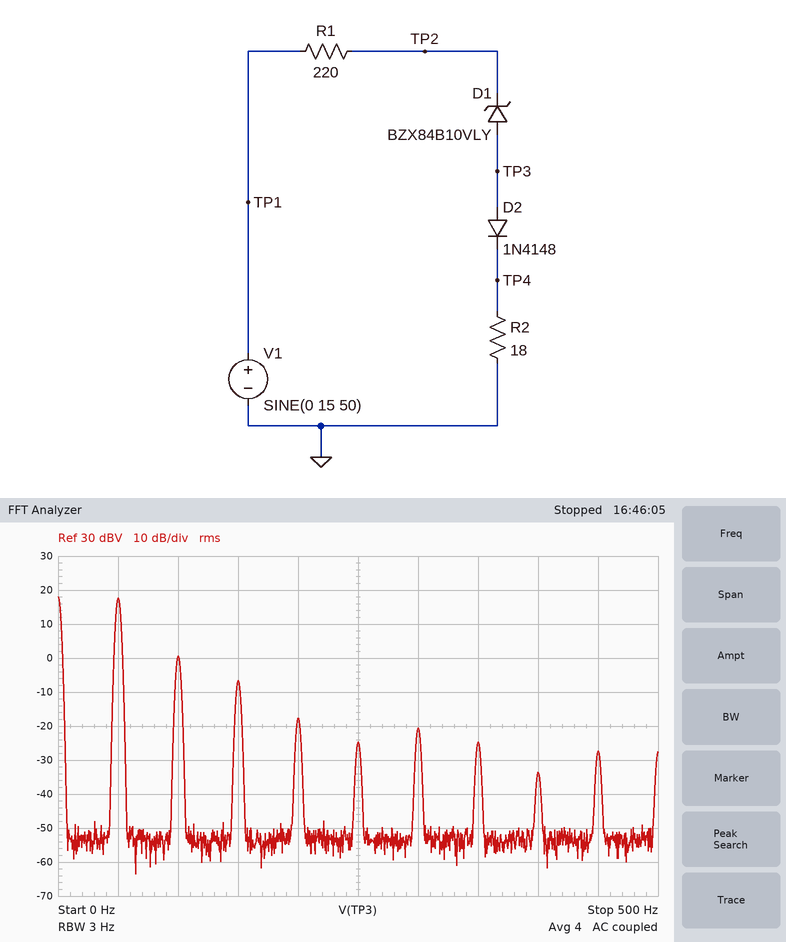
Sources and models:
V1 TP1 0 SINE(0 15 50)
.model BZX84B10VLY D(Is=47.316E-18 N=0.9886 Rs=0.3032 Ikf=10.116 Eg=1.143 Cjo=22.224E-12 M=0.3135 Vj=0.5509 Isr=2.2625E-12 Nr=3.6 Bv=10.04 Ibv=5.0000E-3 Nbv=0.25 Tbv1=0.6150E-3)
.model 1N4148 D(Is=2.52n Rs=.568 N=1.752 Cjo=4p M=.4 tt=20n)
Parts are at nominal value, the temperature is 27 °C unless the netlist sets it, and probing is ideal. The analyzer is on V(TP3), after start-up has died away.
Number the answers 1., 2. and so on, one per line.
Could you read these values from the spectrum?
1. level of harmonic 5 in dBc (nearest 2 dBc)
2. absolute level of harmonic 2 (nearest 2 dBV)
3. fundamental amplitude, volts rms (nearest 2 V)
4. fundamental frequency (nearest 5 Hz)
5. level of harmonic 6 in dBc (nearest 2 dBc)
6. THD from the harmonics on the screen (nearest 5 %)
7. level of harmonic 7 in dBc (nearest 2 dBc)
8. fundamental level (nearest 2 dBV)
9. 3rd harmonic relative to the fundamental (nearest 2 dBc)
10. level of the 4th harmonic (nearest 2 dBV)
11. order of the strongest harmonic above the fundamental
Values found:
1. -42 dBc
2. 0 dBV
3. 8 V
4. 50 Hz
5. -38 dBc
6. 15 %
7. -42 dBc
8. 18 dBV
9. -24 dBc
10. -18 dBV
11. 2
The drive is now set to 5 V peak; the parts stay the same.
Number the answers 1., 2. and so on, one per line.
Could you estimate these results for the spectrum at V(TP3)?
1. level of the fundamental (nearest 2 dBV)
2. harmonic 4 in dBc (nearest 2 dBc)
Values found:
1. 8 dBV
2. -32 dBc
